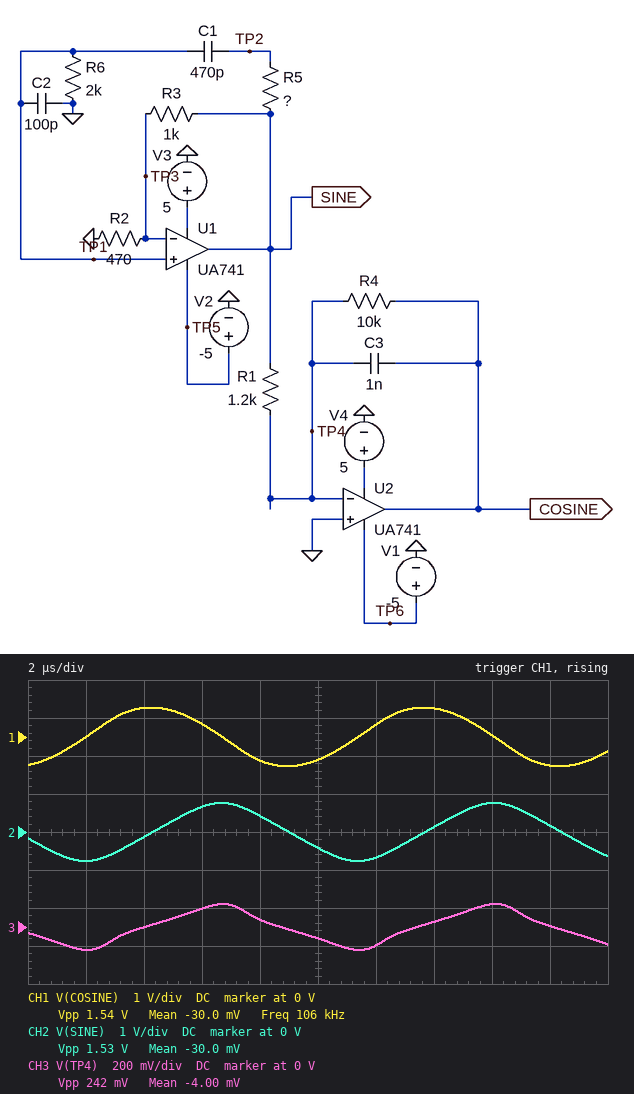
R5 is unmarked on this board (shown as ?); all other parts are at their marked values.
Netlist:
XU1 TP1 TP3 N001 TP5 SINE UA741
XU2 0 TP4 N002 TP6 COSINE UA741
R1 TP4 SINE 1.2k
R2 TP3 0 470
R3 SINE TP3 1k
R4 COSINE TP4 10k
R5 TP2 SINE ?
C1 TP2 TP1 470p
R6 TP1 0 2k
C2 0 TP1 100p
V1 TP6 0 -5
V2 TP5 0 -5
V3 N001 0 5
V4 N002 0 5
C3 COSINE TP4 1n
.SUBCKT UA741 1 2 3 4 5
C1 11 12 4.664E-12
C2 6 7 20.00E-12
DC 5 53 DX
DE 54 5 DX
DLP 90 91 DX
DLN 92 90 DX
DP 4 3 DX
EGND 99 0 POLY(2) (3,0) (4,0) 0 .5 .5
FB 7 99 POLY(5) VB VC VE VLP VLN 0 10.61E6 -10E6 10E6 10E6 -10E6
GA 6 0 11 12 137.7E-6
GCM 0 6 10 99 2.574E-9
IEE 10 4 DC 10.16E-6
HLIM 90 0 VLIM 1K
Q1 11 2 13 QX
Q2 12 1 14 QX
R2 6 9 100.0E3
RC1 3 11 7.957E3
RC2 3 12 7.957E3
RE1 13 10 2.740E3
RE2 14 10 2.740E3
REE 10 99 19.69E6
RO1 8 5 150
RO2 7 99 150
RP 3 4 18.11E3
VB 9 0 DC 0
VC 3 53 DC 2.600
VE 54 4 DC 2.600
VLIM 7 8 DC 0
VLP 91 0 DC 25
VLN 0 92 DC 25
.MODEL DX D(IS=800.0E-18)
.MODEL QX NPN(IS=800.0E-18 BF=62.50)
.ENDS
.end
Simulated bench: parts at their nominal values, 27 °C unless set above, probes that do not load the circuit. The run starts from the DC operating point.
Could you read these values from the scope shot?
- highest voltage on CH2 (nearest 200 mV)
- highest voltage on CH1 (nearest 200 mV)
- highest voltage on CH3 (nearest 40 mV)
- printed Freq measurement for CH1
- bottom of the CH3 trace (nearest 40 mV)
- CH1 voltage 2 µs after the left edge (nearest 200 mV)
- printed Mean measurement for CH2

800 mV
800 mV
120 mV
106 kHz
-120 mV
0 V
-30.0 mV
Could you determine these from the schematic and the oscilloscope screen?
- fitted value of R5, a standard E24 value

2.4 kΩ
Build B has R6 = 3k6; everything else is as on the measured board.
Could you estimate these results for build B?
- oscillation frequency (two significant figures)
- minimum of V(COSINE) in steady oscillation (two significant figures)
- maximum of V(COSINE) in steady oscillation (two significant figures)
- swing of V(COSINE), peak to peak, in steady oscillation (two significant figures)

51 kHz
-2.4 V
2.3 V
4.7 V
